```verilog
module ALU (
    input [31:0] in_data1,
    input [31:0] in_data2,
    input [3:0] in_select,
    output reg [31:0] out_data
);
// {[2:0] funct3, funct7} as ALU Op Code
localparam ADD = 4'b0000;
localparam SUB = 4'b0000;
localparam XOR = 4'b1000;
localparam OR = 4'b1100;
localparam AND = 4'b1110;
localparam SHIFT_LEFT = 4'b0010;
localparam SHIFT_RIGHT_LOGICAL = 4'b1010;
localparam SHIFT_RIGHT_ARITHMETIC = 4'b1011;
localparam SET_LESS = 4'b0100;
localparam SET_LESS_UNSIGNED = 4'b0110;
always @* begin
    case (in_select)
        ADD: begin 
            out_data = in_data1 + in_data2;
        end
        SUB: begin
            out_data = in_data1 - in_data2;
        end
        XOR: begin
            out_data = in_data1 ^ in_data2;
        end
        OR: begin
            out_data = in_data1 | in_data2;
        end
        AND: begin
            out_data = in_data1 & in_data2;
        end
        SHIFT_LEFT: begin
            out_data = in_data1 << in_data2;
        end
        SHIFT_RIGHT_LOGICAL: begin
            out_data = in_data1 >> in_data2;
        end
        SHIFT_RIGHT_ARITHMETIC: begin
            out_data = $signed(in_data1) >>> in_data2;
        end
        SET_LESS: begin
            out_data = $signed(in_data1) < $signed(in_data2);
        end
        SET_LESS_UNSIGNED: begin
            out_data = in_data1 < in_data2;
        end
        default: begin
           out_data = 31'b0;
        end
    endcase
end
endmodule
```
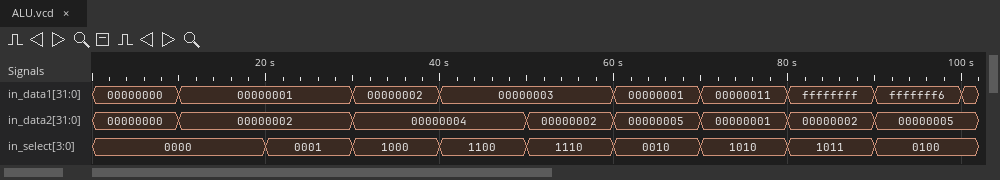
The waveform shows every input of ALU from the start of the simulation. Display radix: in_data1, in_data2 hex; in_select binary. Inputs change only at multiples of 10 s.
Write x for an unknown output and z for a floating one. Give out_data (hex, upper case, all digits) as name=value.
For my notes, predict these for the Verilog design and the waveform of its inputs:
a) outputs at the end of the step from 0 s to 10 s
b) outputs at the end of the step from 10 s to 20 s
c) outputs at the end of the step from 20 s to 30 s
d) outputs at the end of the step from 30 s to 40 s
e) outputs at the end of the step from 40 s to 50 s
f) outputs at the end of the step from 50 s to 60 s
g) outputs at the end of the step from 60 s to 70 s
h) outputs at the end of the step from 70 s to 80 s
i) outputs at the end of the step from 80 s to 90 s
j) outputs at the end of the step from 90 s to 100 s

out_data=00000000
out_data=00000003
out_data=00000000
out_data=00000006
out_data=00000007
out_data=00000002
out_data=00000020
out_data=00000008
out_data=FFFFFFFF
out_data=00000001
